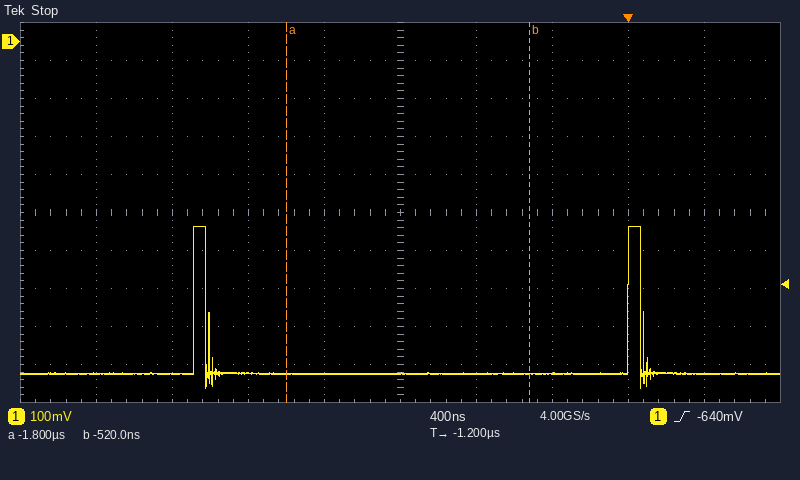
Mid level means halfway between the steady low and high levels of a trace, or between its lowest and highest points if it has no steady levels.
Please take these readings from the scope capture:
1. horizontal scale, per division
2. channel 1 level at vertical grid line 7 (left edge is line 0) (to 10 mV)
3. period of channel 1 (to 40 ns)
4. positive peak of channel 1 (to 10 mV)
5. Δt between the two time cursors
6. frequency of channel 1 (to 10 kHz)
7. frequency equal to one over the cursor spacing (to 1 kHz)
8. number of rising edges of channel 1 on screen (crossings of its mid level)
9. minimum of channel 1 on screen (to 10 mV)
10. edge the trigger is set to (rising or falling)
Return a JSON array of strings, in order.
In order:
["400 ns", "-870 mV", "2.28 µs", "-490 mV", "1.28 µs", "440 kHz", "781 kHz", "2", "-910 mV", "rising"]
